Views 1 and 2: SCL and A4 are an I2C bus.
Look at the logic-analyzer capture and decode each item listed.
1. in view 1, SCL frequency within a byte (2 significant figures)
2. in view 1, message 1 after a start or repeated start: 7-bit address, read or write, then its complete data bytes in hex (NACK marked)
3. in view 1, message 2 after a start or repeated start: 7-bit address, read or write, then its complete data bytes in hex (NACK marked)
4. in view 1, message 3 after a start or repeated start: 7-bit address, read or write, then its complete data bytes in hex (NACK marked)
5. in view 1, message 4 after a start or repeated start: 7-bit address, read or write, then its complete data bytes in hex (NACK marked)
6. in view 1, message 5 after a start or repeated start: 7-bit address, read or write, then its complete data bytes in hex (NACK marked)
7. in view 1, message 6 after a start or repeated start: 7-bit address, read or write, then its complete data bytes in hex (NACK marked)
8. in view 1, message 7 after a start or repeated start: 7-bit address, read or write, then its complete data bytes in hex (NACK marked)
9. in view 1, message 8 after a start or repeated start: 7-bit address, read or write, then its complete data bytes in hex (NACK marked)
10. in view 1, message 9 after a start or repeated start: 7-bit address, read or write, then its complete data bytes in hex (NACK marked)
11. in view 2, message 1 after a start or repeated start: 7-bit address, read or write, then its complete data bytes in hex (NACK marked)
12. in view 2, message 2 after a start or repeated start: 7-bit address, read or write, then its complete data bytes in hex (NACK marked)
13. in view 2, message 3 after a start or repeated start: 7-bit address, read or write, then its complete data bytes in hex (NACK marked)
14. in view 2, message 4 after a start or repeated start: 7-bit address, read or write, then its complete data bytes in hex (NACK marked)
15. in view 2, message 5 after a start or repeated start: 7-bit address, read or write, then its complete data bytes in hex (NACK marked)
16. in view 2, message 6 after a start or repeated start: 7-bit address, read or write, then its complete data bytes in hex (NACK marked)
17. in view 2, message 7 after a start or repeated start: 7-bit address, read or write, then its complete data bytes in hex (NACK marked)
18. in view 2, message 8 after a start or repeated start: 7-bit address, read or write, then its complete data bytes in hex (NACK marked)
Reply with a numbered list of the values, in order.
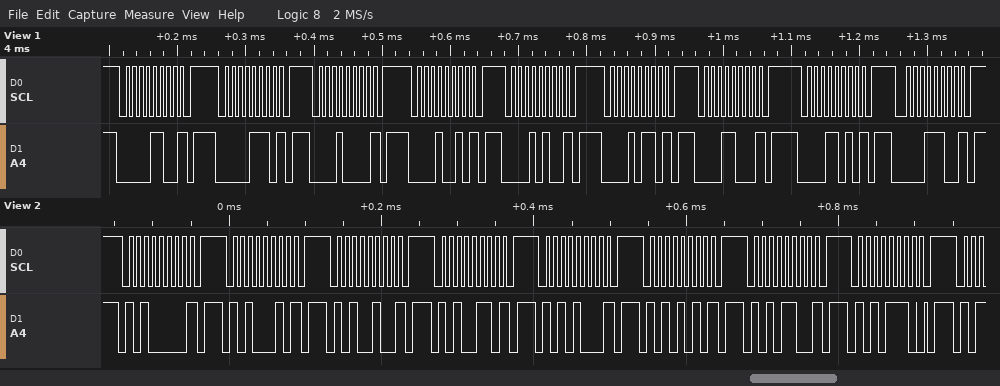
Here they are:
1. 100 kHz
2. 0x06 write NACK
3. 0x07 write NACK
4. 0x08 write NACK
5. 0x09 write NACK
6. 0x0A write NACK
7. 0x0B write NACK
8. 0x0C write NACK
9. 0x0D write NACK
10. 0x0E write NACK
11. 0x50 write NACK
12. 0x51 write NACK
13. 0x52 write NACK
14. 0x53 write NACK
15. 0x54 write NACK
16. 0x55 write NACK
17. 0x56 write NACK
18. 0x57 write
